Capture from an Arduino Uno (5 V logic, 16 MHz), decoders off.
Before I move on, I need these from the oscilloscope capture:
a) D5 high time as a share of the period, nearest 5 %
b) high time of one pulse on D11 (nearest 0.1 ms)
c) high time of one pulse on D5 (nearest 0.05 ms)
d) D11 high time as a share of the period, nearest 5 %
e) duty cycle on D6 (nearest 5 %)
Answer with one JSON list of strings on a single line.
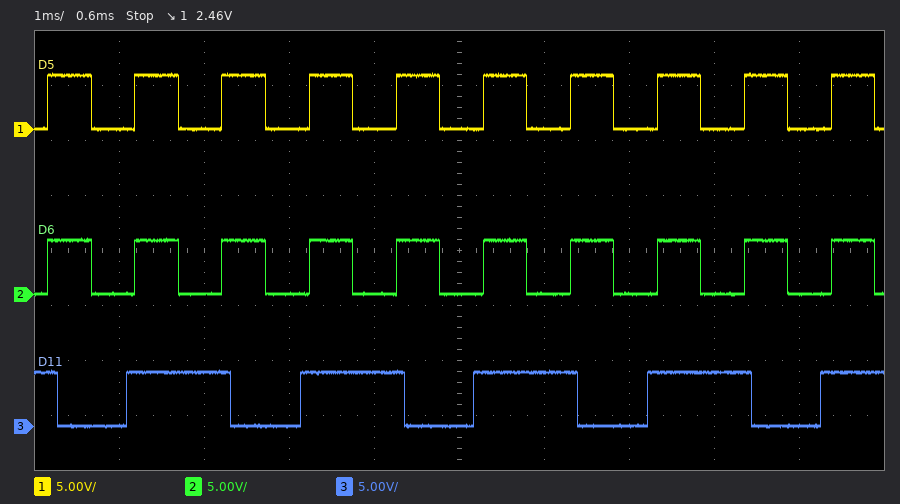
["50 %", "1.2 ms", "0.50 ms", "60 %", "50 %"]
